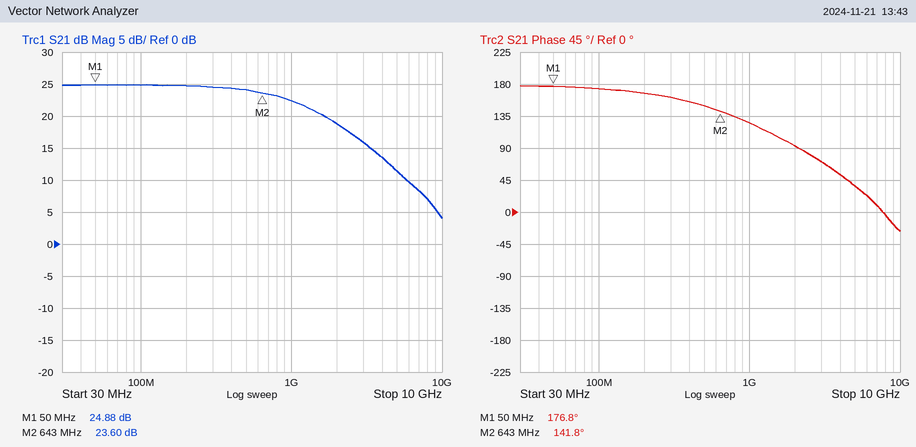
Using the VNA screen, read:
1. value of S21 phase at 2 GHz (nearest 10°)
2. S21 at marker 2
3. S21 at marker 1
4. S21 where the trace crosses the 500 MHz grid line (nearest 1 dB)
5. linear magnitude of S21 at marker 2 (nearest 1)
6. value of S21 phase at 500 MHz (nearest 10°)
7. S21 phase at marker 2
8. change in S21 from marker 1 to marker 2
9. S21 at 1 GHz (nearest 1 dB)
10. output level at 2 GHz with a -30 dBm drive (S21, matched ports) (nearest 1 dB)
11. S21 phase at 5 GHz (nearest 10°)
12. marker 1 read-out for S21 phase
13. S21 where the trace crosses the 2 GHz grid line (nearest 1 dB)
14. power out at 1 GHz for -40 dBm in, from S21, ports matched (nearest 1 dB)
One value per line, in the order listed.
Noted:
90°
23.60 dB
24.88 dB
24 dB
15
150°
141.8°
-1.28 dB
22 dB
-11 dBm
40°
176.8°
19 dB
-18 dBm
